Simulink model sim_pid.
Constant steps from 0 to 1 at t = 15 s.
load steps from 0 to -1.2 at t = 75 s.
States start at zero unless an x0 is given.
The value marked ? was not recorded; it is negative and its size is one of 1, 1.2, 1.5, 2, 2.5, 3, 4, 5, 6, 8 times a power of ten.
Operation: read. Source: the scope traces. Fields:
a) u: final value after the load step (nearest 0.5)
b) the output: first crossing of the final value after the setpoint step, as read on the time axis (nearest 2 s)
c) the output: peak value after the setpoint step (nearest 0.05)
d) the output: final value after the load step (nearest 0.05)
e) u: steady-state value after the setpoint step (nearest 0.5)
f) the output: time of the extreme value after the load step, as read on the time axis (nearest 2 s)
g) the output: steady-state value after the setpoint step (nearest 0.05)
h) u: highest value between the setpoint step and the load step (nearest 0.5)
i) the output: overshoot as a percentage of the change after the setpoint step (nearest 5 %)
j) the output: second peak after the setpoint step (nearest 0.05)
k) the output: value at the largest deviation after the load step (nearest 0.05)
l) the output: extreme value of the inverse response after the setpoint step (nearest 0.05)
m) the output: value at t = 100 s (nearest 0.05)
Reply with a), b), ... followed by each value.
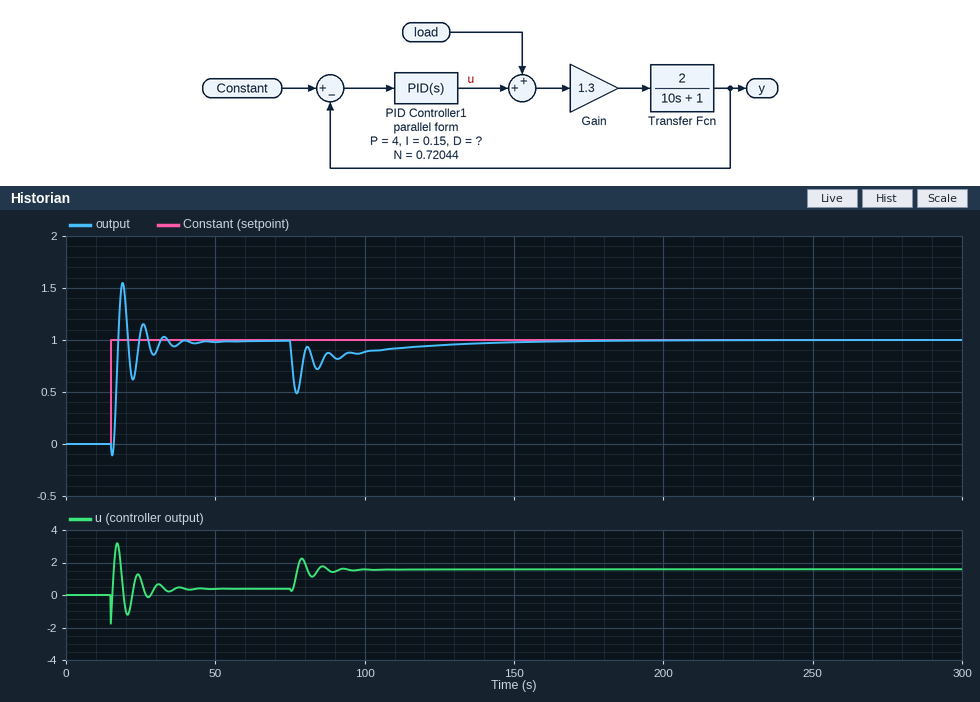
a) 1.5
b) 18 s
c) 1.55
d) 1.00
e) 0.5
f) 78 s
g) 1.00
h) 3.0
i) 55 %
j) 1.15
k) 0.50
l) -0.10
m) 0.90
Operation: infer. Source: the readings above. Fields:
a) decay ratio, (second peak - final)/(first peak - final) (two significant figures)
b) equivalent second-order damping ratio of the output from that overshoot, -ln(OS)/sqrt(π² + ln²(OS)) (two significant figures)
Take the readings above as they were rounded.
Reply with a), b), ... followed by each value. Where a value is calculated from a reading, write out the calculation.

a) (1.15 - 1) / (1.55 - 1) = 0.27
b) ln(0.55) = -0.598; 0.598 / sqrt(9.870 + 0.357) = 0.19
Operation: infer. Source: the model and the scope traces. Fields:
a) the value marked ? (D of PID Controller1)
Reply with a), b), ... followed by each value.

a) -8
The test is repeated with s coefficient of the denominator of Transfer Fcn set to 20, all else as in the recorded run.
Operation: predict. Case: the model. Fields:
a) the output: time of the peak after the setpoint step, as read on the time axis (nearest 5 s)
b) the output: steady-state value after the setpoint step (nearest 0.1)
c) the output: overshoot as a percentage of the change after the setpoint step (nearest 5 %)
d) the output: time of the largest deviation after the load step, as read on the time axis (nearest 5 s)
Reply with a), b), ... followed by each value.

a) 20 s
b) 1.0
c) 25 %
d) 80 s
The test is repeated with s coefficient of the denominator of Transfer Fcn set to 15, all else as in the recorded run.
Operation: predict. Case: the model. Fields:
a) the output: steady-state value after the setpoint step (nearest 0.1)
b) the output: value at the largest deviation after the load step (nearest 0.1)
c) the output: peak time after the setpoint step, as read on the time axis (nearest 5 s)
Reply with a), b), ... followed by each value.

a) 1.0
b) 0.6
c) 20 s
